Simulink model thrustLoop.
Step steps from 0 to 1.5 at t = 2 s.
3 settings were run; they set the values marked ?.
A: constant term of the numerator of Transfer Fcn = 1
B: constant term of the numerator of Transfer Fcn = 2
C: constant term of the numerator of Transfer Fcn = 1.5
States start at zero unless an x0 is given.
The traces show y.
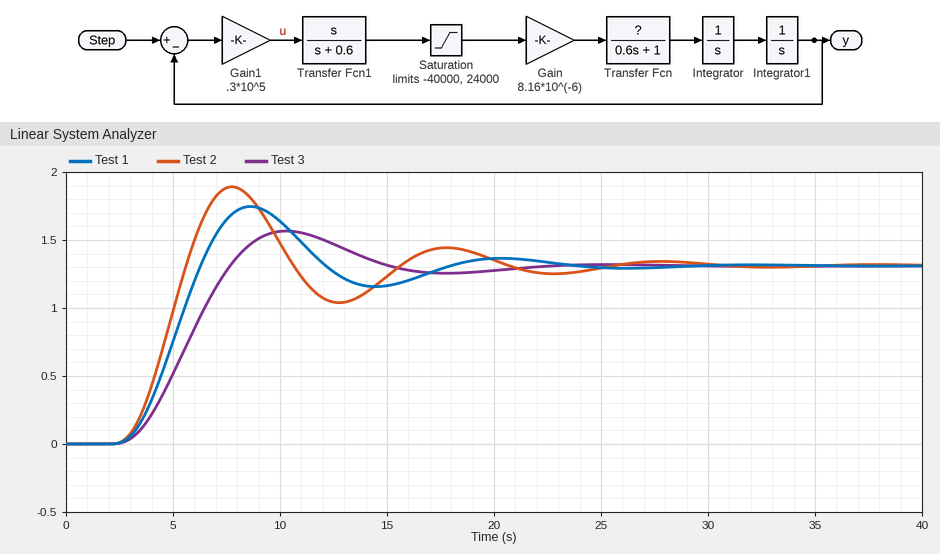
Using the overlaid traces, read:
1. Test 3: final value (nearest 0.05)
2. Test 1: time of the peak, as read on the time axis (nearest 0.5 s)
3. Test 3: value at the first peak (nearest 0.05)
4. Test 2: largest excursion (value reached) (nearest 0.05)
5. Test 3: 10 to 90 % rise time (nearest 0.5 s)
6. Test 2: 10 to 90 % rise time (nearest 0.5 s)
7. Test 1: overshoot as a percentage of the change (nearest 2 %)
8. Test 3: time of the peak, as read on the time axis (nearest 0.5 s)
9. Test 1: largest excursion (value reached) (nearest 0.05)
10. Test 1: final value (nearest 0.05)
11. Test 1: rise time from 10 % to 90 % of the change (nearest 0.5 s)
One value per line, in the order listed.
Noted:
1.30
8.5 s
1.55
1.90
3.5 s
2.0 s
34 %
10.5 s
1.75
1.30
2.5 s
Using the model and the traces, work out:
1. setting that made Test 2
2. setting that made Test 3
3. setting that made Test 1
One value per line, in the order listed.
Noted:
B
A
C
